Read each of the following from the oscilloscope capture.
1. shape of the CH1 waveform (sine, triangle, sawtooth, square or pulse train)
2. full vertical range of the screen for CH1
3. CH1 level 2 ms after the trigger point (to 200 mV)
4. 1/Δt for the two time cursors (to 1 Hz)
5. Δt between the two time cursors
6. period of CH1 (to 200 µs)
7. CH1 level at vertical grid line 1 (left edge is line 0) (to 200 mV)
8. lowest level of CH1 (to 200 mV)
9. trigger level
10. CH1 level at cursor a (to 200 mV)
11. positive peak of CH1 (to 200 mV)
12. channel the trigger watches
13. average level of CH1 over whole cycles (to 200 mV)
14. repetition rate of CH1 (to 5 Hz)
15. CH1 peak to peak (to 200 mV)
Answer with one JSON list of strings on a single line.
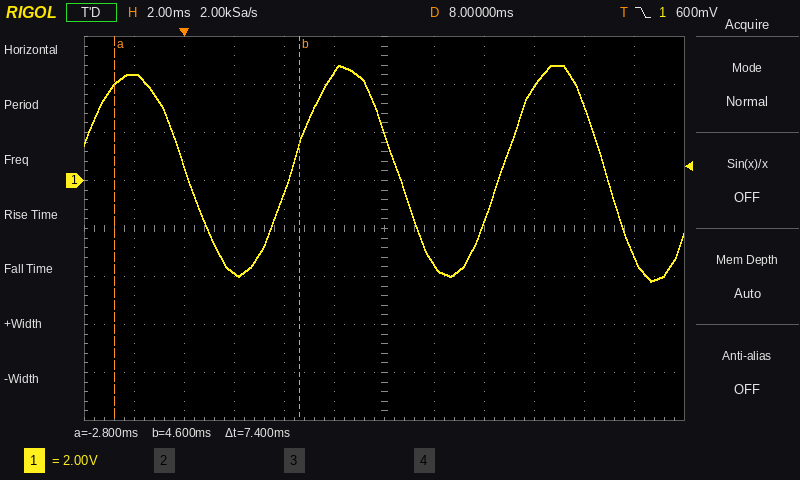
["sine", "16 V", "-3.8 V", "135 Hz", "7.4 ms", "8.4 ms", "4.4 V", "-4.2 V", "600 mV", "4.0 V", "4.8 V", "CH1", "400 mV", "120 Hz", "9.0 V"]
